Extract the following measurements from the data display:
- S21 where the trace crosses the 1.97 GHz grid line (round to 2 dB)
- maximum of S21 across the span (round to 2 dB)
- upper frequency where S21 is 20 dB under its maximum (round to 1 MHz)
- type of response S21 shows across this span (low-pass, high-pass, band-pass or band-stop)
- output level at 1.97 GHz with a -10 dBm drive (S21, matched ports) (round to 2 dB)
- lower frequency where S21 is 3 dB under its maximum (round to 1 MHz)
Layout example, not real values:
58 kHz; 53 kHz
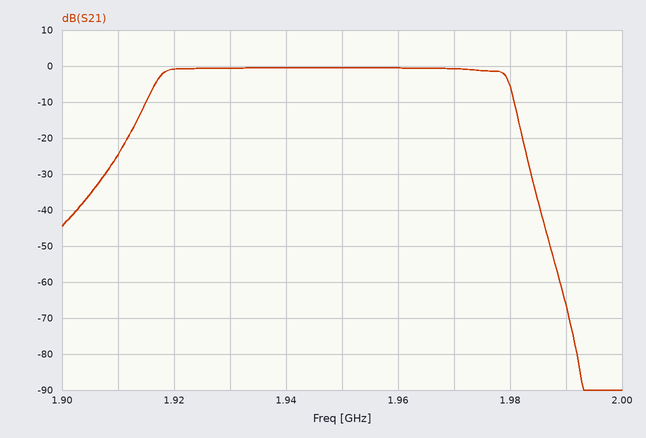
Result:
0 dB; 0 dB; 1.982 GHz; band-pass; -10 dBm; 1.917 GHz
